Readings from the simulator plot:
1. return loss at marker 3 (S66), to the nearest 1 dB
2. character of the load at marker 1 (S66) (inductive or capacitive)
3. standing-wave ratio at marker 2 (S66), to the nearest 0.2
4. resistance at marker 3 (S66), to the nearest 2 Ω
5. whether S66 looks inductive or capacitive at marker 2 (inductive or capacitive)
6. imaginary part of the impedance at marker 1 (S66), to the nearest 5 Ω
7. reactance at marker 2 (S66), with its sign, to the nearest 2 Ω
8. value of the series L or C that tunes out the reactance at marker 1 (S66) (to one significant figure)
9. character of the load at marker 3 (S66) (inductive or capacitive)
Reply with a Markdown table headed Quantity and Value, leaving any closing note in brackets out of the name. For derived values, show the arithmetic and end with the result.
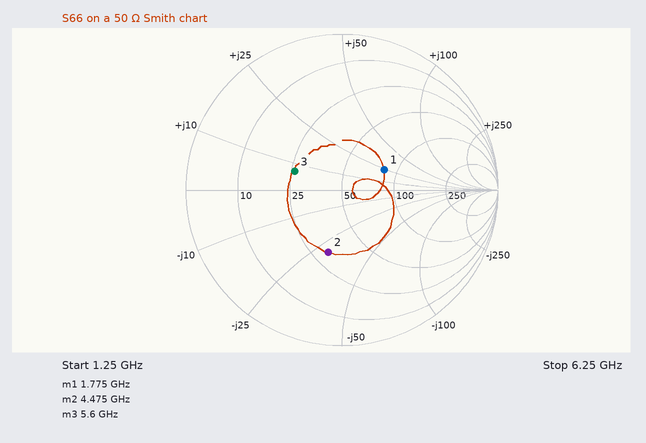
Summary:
| Quantity | Value |
|---|---|
| return loss at marker 3 (S66), to the nearest 1 dB | 10 dB |
| character of the load at marker 1 (S66) | inductive |
| standing-wave ratio at marker 2 (S66), to the nearest 0.2 | 2.4 |
| resistance at marker 3 (S66), to the nearest 2 Ω | 26 Ω |
| whether S66 looks inductive or capacitive at marker 2 | capacitive |
| imaginary part of the impedance at marker 1 (S66), to the nearest 5 Ω | +25 Ω |
| reactance at marker 2 (S66), with its sign, to the nearest 2 Ω | -30 Ω |
| value of the series L or C that tunes out the reactance at marker 1 (S66) | C = 1/(2π × 1.775 GHz × 25 Ω) ≈ 4 pF |
| character of the load at marker 3 (S66) | inductive |
